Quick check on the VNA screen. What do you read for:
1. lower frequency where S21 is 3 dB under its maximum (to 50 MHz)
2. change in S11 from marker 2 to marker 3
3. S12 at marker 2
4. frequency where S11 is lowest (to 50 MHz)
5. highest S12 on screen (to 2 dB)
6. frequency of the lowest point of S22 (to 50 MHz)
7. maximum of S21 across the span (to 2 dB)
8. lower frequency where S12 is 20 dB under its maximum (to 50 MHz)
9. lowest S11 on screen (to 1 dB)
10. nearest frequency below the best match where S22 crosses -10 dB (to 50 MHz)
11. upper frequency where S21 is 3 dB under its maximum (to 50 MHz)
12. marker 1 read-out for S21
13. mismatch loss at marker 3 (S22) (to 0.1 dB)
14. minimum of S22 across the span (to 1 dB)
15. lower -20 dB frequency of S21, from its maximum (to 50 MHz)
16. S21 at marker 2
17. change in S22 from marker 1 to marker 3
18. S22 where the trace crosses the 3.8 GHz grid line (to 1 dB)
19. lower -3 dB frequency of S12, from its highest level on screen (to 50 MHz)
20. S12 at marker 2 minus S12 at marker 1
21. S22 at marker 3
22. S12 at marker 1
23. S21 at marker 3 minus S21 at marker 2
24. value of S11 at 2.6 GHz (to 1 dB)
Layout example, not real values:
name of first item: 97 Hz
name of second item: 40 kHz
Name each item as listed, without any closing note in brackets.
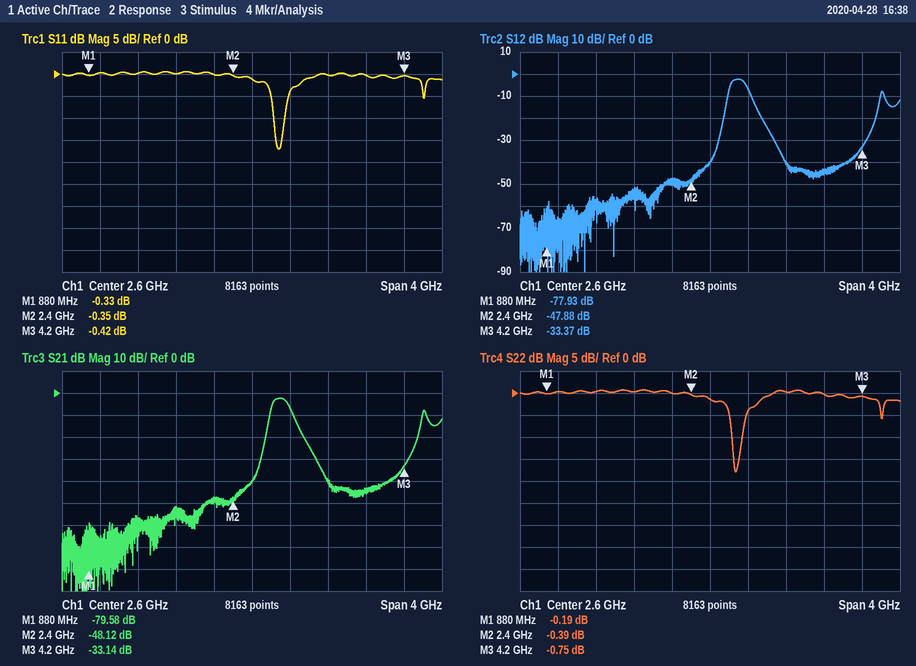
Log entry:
lower frequency where S21 is 3 dB under its maximum: 2.80 GHz
change in S11 from marker 2 to marker 3: -0.07 dB
S12 at marker 2: -47.88 dB
frequency where S11 is lowest: 2.90 GHz
highest S12 on screen: -2 dB
frequency of the lowest point of S22: 2.85 GHz
maximum of S21 across the span: -2 dB
lower frequency where S12 is 20 dB under its maximum: 2.75 GHz
lowest S11 on screen: -17 dB
nearest frequency below the best match where S22 crosses -10 dB: 2.85 GHz
upper frequency where S21 is 3 dB under its maximum: 3.00 GHz
marker 1 read-out for S21: -79.58 dB
mismatch loss at marker 3 (S22): 8.0 dB
minimum of S22 across the span: -18 dB
lower -20 dB frequency of S21, from its maximum: 2.75 GHz
S21 at marker 2: -48.12 dB
change in S22 from marker 1 to marker 3: -0.56 dB
S22 where the trace crosses the 3.8 GHz grid line: 0 dB
lower -3 dB frequency of S12, from its highest level on screen: 2.80 GHz
S12 at marker 2 minus S12 at marker 1: 30.05 dB
S22 at marker 3: -0.75 dB
S12 at marker 1: -77.93 dB
S21 at marker 3 minus S21 at marker 2: 14.98 dB
value of S11 at 2.6 GHz: -1 dB
